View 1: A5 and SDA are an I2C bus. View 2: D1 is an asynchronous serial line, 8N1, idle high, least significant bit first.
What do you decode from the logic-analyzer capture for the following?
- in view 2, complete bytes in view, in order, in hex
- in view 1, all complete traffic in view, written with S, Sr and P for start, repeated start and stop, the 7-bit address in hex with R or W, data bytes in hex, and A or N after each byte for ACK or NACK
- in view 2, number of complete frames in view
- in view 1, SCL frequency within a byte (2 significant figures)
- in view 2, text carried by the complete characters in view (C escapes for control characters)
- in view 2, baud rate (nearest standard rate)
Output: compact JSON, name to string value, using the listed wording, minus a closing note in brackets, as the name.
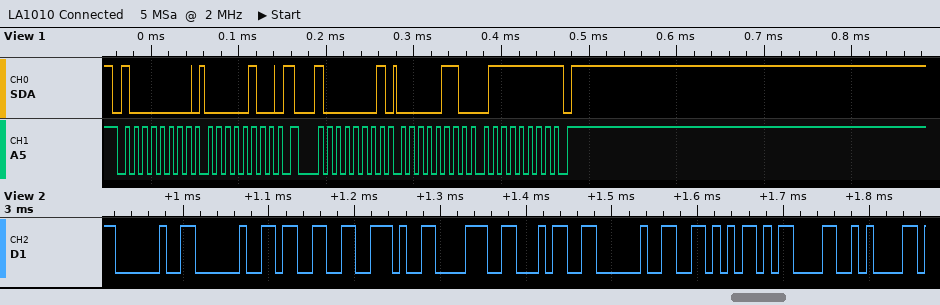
{"in view 2, complete bytes in view, in order, in hex": "20 20 33 2E 38 34 20 56 0D 0A", "in view 1, all complete traffic in view, written with S, Sr and P for start, repeated start and stop, the 7-bit address in hex with R or W, data bytes in hex, and A or N after each byte for ACK or NACK": "S 40W A 04 A Sr 40R A 06 A 7F N P", "in view 2, number of complete frames in view": "10", "in view 1, SCL frequency within a byte": "100 kHz", "in view 2, text carried by the complete characters in view": "\"  3.84 V\\r\\n\"", "in view 2, baud rate": "115200 baud"}
